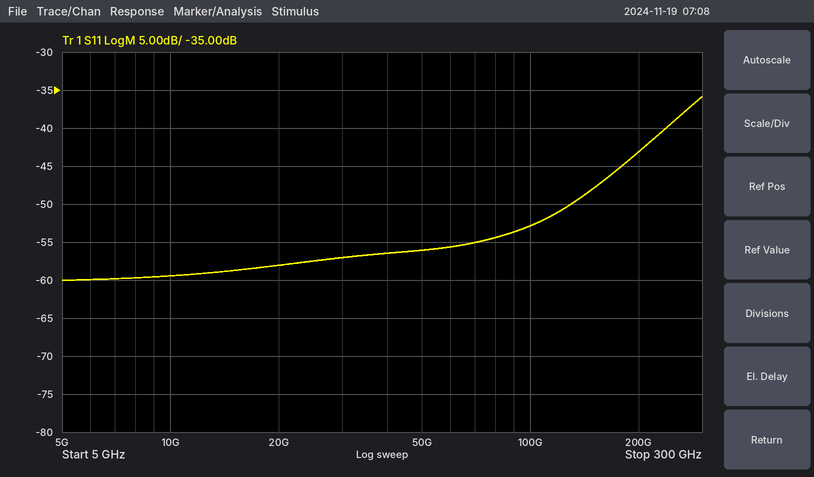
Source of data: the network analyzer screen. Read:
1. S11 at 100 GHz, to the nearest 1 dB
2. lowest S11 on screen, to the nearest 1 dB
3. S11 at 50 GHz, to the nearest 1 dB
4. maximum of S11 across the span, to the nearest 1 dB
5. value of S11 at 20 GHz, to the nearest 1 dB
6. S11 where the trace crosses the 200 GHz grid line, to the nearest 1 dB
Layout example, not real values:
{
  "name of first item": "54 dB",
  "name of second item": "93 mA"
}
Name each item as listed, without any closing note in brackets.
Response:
{
  "S11 at 100 GHz, to the nearest 1 dB": "-53 dB",
  "lowest S11 on screen, to the nearest 1 dB": "-60 dB",
  "S11 at 50 GHz, to the nearest 1 dB": "-56 dB",
  "maximum of S11 across the span, to the nearest 1 dB": "-36 dB",
  "value of S11 at 20 GHz, to the nearest 1 dB": "-58 dB",
  "S11 where the trace crosses the 200 GHz grid line, to the nearest 1 dB": "-43 dB"
}
